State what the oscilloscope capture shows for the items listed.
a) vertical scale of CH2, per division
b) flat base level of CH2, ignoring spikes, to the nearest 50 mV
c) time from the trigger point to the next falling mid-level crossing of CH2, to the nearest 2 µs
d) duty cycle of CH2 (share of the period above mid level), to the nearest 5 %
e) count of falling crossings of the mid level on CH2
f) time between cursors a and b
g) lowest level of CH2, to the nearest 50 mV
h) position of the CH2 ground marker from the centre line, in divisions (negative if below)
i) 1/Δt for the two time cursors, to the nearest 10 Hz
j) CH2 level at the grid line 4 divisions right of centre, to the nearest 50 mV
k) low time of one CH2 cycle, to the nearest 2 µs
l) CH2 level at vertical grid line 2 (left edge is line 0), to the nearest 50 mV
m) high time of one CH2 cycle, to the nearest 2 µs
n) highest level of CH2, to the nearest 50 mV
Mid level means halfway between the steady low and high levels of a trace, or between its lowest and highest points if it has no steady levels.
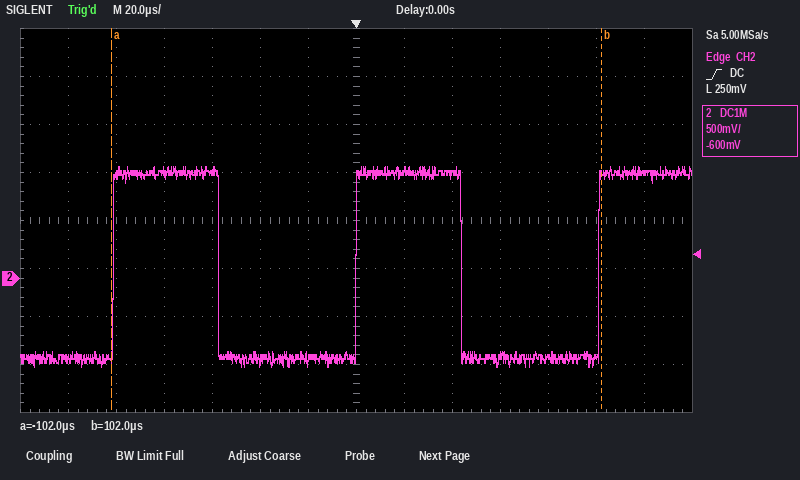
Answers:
500 mV
-850 mV
44 µs
45 %
2
204 µs
-900 mV
-1.2 div
4.90 kHz
-800 mV
58 µs
1.10 V
44 µs
1.15 V
